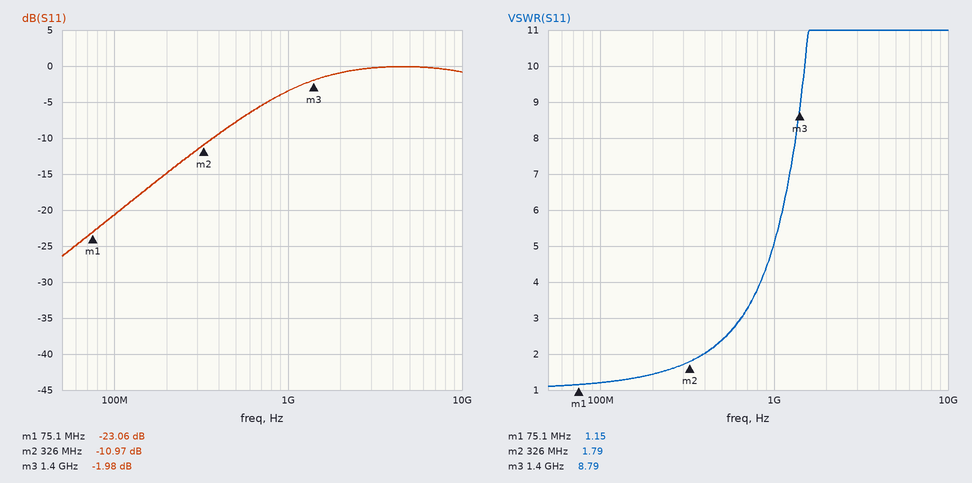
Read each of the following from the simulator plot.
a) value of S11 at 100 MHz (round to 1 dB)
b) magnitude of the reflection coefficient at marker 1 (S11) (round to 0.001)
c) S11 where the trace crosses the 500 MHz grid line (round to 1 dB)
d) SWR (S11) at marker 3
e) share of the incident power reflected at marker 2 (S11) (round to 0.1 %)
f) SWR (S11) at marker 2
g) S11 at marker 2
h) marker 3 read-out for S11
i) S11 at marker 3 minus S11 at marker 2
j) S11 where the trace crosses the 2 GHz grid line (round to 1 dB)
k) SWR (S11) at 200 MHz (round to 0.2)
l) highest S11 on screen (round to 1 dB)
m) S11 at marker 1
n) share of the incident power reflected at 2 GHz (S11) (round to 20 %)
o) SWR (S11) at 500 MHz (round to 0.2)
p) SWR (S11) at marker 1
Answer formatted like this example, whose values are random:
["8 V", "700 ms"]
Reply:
["-21 dB", "0.070", "-8 dB", "8.79", "8.0 %", "1.79", "-10.97 dB", "-1.98 dB", "8.99 dB", "-1 dB", "1.4", "0 dB", "-23.06 dB", "80 %", "2.4", "1.15"]
